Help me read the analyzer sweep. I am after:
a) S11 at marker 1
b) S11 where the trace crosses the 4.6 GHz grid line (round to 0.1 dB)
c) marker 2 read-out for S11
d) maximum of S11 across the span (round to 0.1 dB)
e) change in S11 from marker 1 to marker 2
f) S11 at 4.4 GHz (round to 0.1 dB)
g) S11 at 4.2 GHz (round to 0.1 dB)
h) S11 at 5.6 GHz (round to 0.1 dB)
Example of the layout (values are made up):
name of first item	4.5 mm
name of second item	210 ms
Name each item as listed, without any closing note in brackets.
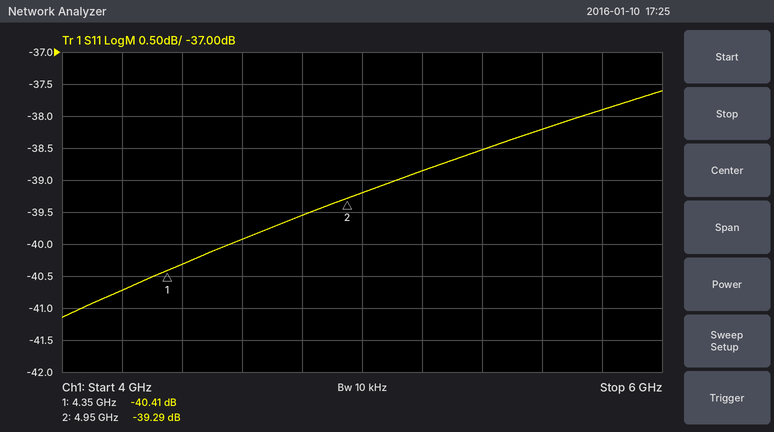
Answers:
S11 at marker 1	-40.41 dB
S11 where the trace crosses the 4.6 GHz grid line	-39.9 dB
marker 2 read-out for S11	-39.29 dB
maximum of S11 across the span	-37.6 dB
change in S11 from marker 1 to marker 2	1.12 dB
S11 at 4.4 GHz	-40.3 dB
S11 at 4.2 GHz	-40.7 dB
S11 at 5.6 GHz	-38.2 dB
